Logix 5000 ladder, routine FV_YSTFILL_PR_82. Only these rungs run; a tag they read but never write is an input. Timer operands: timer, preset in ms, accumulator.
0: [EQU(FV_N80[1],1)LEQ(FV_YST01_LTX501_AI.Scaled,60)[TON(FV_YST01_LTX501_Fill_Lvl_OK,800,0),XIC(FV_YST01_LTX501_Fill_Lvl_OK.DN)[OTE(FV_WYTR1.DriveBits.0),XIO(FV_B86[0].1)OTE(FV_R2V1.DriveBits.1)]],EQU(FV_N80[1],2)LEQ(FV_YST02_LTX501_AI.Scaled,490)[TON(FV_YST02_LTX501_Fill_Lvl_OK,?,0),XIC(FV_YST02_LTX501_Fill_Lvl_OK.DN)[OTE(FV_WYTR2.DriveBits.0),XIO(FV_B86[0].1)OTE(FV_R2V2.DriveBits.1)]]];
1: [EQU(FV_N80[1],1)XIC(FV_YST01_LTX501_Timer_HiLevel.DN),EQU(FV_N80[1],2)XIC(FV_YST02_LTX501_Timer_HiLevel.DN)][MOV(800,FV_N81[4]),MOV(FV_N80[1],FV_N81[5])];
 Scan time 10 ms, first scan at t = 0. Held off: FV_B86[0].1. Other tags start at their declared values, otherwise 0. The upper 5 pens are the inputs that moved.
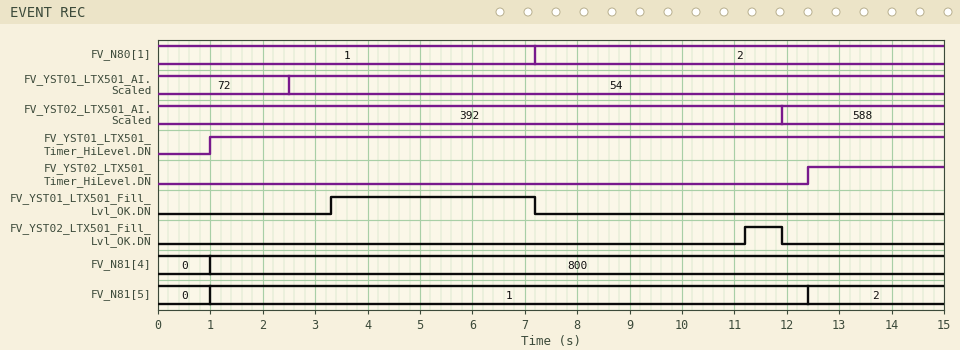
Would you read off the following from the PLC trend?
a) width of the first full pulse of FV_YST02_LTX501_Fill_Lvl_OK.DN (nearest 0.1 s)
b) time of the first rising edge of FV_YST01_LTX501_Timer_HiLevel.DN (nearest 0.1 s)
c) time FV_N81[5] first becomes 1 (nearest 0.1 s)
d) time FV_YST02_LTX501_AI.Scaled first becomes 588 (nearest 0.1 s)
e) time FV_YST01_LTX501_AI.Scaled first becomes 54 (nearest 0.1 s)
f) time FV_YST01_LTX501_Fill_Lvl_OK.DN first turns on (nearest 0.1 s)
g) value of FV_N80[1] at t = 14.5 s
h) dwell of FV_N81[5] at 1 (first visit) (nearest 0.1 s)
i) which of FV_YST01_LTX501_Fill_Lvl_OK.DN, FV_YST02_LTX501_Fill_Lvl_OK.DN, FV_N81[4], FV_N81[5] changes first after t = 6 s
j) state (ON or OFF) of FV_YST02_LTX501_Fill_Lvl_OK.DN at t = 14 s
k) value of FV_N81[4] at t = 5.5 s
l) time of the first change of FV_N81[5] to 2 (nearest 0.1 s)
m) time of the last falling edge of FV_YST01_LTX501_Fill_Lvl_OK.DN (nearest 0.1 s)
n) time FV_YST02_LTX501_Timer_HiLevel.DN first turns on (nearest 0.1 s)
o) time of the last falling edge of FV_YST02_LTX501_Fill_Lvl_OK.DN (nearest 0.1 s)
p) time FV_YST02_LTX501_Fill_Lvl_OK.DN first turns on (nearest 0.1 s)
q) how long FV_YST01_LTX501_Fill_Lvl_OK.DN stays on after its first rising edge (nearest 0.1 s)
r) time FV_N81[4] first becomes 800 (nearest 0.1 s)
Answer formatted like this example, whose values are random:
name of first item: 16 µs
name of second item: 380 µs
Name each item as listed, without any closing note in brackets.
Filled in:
width of the first full pulse of FV_YST02_LTX501_Fill_Lvl_OK.DN: 0.7 s
time of the first rising edge of FV_YST01_LTX501_Timer_HiLevel.DN: 1.0 s
time FV_N81[5] first becomes 1: 1.0 s
time FV_YST02_LTX501_AI.Scaled first becomes 588: 11.9 s
time FV_YST01_LTX501_AI.Scaled first becomes 54: 2.5 s
time FV_YST01_LTX501_Fill_Lvl_OK.DN first turns on: 3.3 s
value of FV_N80[1] at t = 14.5 s: 2
dwell of FV_N81[5] at 1 (first visit): 11.4 s
which of FV_YST01_LTX501_Fill_Lvl_OK.DN, FV_YST02_LTX501_Fill_Lvl_OK.DN, FV_N81[4], FV_N81[5] changes first after t = 6 s: FV_YST01_LTX501_Fill_Lvl_OK.DN
state (ON or OFF) of FV_YST02_LTX501_Fill_Lvl_OK.DN at t = 14 s: OFF
value of FV_N81[4] at t = 5.5 s: 800
time of the first change of FV_N81[5] to 2: 12.4 s
time of the last falling edge of FV_YST01_LTX501_Fill_Lvl_OK.DN: 7.2 s
time FV_YST02_LTX501_Timer_HiLevel.DN first turns on: 12.4 s
time of the last falling edge of FV_YST02_LTX501_Fill_Lvl_OK.DN: 11.9 s
time FV_YST02_LTX501_Fill_Lvl_OK.DN first turns on: 11.2 s
how long FV_YST01_LTX501_Fill_Lvl_OK.DN stays on after its first rising edge: 3.9 s
time FV_N81[4] first becomes 800: 1.0 s
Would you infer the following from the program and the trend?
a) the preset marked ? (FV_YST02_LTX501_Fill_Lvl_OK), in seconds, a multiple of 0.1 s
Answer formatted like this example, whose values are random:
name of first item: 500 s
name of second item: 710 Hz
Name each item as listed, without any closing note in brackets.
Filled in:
the preset marked ? (FV_YST02_LTX501_Fill_Lvl_OK), in seconds, a multiple of 0.1 s: 4.0 s
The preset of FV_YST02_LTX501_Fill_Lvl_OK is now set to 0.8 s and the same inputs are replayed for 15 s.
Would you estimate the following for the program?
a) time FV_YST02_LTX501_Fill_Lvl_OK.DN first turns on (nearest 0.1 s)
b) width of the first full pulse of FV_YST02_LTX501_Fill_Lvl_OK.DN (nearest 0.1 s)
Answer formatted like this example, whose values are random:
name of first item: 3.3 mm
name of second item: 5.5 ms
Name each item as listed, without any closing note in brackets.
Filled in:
time FV_YST02_LTX501_Fill_Lvl_OK.DN first turns on: 8.0 s
width of the first full pulse of FV_YST02_LTX501_Fill_Lvl_OK.DN: 3.9 s
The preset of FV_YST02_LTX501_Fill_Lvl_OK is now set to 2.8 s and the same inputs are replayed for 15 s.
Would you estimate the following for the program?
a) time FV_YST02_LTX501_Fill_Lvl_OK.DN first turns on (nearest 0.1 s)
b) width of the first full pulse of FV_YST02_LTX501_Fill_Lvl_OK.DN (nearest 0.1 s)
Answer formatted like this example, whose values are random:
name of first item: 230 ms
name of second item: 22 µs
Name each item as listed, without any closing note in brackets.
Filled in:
time FV_YST02_LTX501_Fill_Lvl_OK.DN first turns on: 10.0 s
width of the first full pulse of FV_YST02_LTX501_Fill_Lvl_OK.DN: 1.9 s
